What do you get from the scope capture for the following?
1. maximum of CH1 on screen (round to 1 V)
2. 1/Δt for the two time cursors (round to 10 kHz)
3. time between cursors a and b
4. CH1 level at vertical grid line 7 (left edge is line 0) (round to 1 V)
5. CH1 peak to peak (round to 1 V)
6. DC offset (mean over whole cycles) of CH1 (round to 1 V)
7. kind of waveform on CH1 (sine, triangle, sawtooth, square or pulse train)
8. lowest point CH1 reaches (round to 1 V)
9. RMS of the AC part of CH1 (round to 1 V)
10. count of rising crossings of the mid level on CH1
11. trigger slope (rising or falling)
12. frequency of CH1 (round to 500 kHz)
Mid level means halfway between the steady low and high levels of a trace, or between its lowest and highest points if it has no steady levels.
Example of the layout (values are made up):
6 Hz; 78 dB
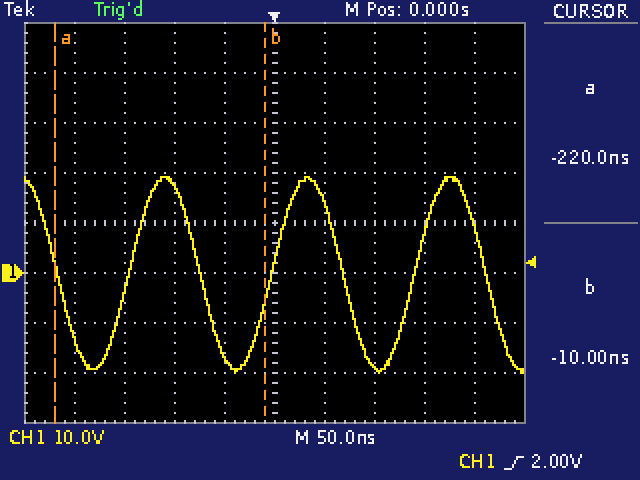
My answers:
19 V; 4.76 MHz; 210 ns; -19 V; 39 V; 0 V; sine; -20 V; 14 V; 3; rising; 7.0 MHz
